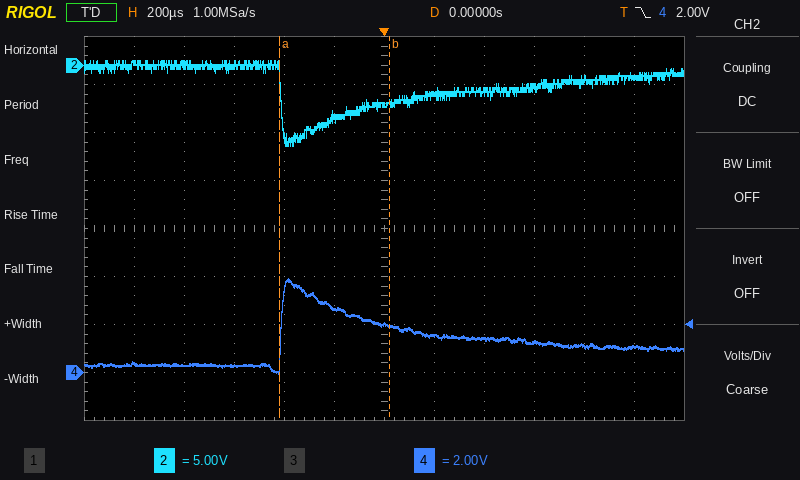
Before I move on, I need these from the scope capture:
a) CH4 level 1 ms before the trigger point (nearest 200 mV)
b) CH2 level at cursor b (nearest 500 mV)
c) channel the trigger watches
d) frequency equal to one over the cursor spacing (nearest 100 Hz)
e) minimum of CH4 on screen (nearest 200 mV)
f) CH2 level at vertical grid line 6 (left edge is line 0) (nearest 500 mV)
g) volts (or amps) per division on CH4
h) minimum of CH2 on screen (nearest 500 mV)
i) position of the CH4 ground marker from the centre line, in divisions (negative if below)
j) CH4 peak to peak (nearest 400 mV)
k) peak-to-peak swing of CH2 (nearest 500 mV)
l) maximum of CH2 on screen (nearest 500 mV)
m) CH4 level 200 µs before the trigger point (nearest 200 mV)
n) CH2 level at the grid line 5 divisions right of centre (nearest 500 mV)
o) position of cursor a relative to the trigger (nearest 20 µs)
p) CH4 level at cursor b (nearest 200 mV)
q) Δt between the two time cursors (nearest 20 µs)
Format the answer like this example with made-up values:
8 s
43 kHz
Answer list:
400 mV
-4.0 V
CH4
2.3 kHz
0.0 V
-4.0 V
2 V
-8.5 V
-3.0 div
4.0 V
9.0 V
500 mV
2.6 V
-1.5 V
-420 µs
2.0 V
440 µs
